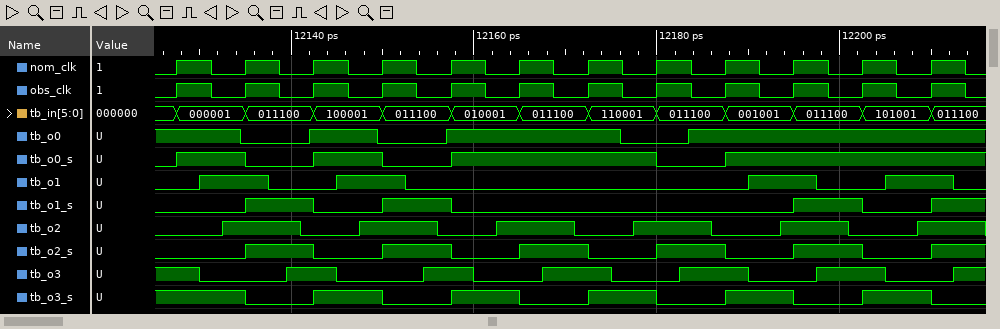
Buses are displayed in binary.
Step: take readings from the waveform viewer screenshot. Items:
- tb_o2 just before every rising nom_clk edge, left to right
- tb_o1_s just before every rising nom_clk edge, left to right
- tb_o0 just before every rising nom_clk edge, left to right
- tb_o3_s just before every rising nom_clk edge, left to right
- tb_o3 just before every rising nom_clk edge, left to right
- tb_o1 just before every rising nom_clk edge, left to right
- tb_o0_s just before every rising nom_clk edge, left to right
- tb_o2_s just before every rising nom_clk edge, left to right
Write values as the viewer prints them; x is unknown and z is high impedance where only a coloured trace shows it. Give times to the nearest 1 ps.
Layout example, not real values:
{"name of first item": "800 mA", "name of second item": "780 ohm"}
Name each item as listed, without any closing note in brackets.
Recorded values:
{"tb_o2 just before every rising nom_clk edge, left to right": "0 1 0 1 0 1 0 1 0 1 0 1", "tb_o1_s just before every rising nom_clk edge, left to right": "0 0 1 0 1 0 0 0 0 0 1 0", "tb_o0 just before every rising nom_clk edge, left to right": "1 0 1 0 1 1 1 0 1 1 1 1", "tb_o3_s just before every rising nom_clk edge, left to right": "1 1 0 1 0 1 0 1 0 1 0 1", "tb_o3 just before every rising nom_clk edge, left to right": "1 0 1 0 1 0 1 0 1 0 1 0", "tb_o1 just before every rising nom_clk edge, left to right": "0 1 0 1 0 0 0 0 0 1 0 1", "tb_o0_s just before every rising nom_clk edge, left to right": "0 1 0 1 0 1 1 1 0 1 1 1", "tb_o2_s just before every rising nom_clk edge, left to right": "0 0 1 0 1 0 1 0 1 0 1 0"}
